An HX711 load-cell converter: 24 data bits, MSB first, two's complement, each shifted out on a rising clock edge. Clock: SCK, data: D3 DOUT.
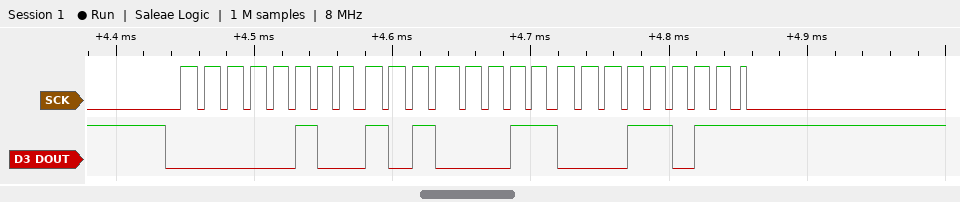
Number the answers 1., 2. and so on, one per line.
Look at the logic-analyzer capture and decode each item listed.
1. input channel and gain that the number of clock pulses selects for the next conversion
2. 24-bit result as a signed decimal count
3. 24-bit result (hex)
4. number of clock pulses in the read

1. channel A, gain 128
2. 303899
3. 0x04A31B
4. 25
